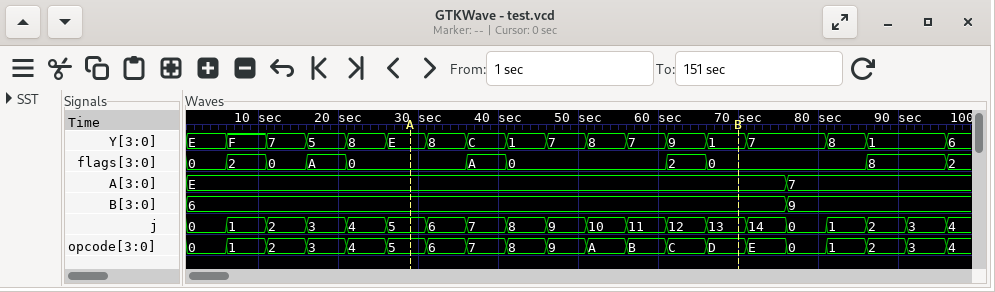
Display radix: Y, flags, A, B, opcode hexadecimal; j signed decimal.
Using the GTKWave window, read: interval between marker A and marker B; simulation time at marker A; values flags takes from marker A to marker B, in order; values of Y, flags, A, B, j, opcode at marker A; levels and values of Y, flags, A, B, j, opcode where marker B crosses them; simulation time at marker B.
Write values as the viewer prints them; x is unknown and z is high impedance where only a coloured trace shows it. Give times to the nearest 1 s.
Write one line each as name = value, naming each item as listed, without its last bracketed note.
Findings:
interval between marker A and marker B = 41 s
simulation time at marker A = 29 s
values flags takes from marker A to marker B, in order = 0, A, 0, 2, 0
values of Y, flags, A, B, j, opcode at marker A = Y=E, flags=0, A=E, B=6, j=5, opcode=5
levels and values of Y, flags, A, B, j, opcode where marker B crosses them = Y=1, flags=0, A=E, B=6, j=13, opcode=D
simulation time at marker B = 70 s
